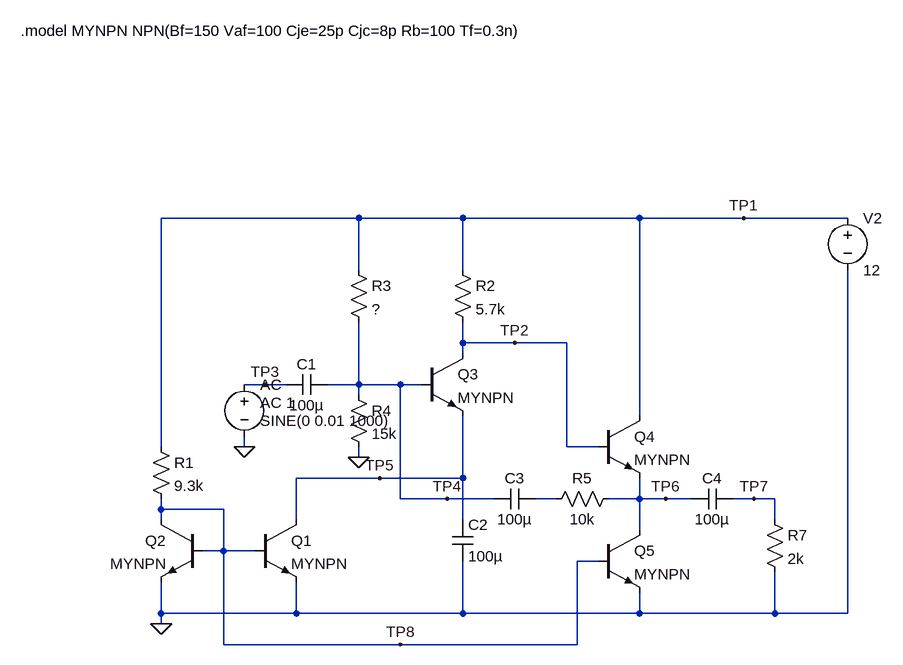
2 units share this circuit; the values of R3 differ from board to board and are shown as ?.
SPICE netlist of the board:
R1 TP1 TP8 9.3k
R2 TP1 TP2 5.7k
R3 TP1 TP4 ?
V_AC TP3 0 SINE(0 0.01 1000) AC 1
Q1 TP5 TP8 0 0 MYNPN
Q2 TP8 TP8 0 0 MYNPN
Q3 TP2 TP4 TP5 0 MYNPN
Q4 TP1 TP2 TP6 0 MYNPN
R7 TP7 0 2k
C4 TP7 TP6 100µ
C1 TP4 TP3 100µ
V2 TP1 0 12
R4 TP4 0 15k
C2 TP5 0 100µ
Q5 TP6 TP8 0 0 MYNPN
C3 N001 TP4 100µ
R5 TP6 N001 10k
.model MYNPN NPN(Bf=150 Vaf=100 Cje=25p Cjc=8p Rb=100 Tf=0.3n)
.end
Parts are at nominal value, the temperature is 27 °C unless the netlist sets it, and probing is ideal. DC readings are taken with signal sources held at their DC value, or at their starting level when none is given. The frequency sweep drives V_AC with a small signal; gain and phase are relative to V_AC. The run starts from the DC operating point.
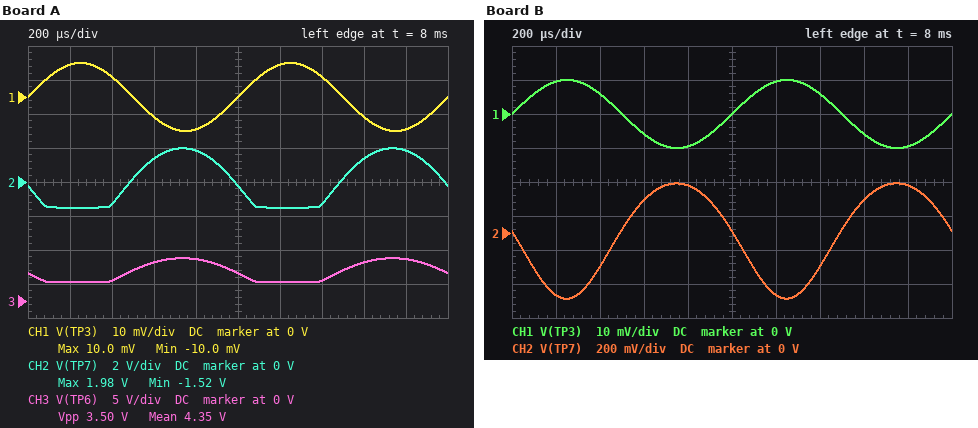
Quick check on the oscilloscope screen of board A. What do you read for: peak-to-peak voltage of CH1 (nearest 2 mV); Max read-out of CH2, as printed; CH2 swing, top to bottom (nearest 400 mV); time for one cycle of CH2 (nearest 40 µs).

20 mV
1.98 V
3.6 V
1.00 ms
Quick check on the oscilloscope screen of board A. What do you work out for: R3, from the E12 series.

27 kΩ
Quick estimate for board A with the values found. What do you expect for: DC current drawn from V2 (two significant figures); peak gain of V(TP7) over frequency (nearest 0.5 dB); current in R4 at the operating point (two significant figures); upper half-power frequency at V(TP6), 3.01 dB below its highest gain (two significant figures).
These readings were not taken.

3.9 mA
47.5 dB
280 µA
770 kHz
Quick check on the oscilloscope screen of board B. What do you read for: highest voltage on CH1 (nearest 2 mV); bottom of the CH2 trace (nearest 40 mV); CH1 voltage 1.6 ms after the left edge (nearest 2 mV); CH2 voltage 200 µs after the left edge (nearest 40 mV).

10 mV
-400 mV
-6 mV
-360 mV
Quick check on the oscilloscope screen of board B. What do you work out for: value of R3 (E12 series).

220 kΩ
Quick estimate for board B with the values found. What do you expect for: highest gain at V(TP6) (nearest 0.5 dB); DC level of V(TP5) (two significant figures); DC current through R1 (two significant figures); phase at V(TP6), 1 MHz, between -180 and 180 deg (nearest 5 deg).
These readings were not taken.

30.5 dB
28 mV
1.2 mA
155 deg
